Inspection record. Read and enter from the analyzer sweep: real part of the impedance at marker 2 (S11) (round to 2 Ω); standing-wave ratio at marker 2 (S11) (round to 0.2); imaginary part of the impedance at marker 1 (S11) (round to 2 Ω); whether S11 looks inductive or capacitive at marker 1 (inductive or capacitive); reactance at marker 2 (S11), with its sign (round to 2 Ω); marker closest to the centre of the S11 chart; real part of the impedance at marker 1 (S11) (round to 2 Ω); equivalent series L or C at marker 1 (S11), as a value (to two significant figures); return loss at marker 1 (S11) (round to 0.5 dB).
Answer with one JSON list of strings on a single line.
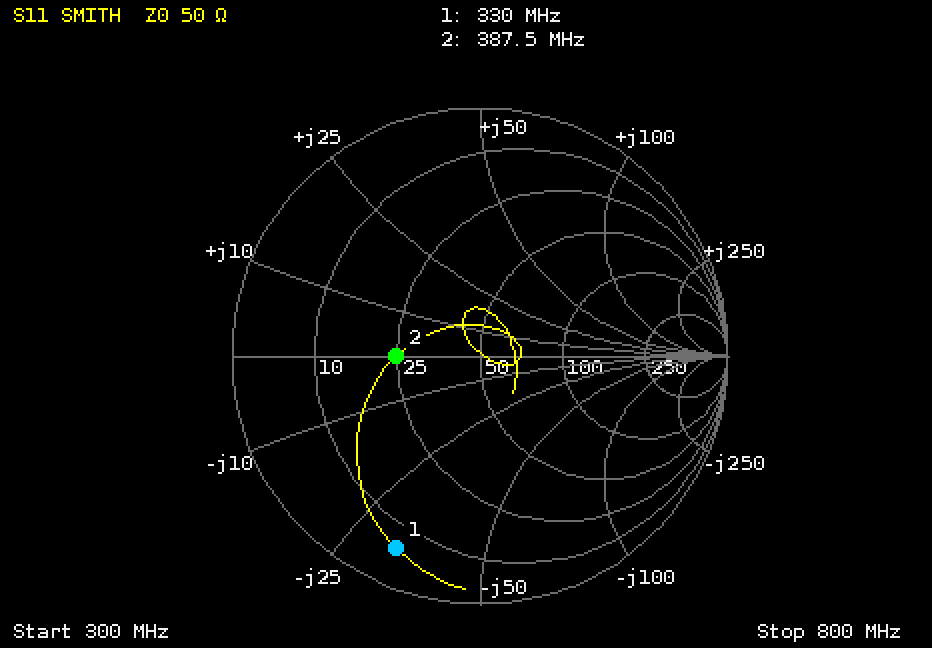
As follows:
["24 Ω", "2.0", "-32 Ω", "capacitive", "0 Ω", "marker 2", "6 Ω", "15 pF", "1.5 dB"]
